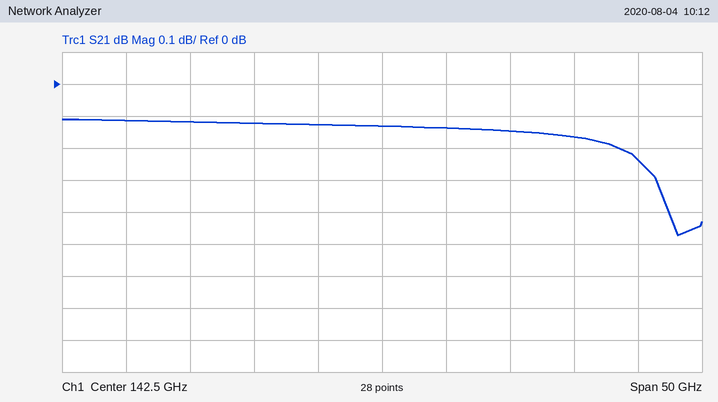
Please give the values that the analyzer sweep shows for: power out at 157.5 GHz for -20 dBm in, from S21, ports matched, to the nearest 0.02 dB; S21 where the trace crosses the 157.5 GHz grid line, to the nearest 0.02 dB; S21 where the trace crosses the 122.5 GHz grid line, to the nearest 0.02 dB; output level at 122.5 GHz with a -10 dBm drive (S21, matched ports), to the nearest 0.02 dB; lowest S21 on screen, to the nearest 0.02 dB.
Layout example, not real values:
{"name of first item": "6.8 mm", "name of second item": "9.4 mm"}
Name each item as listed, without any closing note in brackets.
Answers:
{"power out at 157.5 GHz for -20 dBm in, from S21, ports matched, to the nearest 0.02 dB": "-20.16 dBm", "S21 where the trace crosses the 157.5 GHz grid line, to the nearest 0.02 dB": "-0.16 dB", "S21 where the trace crosses the 122.5 GHz grid line, to the nearest 0.02 dB": "-0.12 dB", "output level at 122.5 GHz with a -10 dBm drive (S21, matched ports), to the nearest 0.02 dB": "-10.12 dBm", "lowest S21 on screen, to the nearest 0.02 dB": "-0.48 dB"}
